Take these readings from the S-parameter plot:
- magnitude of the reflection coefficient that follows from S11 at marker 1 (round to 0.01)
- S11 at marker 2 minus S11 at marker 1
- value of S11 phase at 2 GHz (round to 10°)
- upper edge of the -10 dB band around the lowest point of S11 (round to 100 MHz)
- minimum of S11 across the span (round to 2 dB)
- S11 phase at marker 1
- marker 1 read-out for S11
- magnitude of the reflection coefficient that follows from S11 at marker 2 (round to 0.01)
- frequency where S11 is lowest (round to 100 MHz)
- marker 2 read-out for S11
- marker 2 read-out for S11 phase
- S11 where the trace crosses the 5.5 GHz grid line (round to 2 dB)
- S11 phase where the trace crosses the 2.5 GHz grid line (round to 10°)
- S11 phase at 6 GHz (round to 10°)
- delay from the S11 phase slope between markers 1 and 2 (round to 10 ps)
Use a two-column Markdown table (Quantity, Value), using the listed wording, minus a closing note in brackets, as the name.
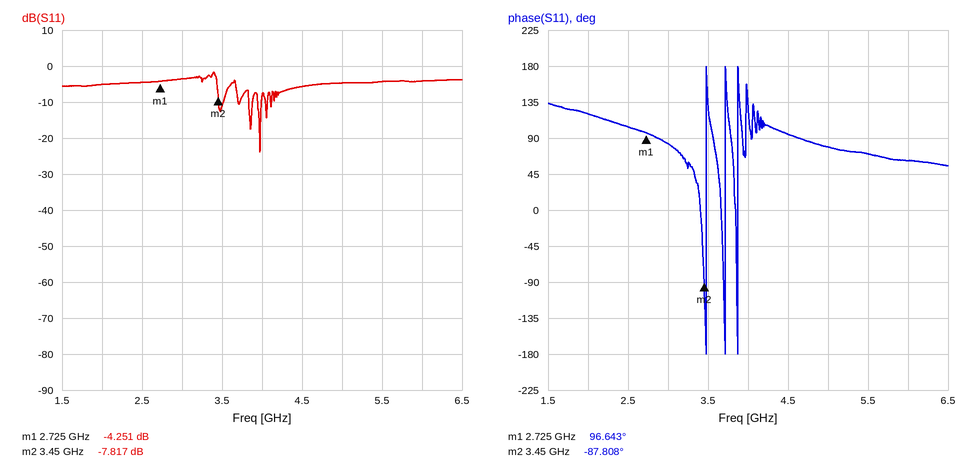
| Quantity | Value |
|---|---|
| magnitude of the reflection coefficient that follows from S11 at marker 1 | 0.61 |
| S11 at marker 2 minus S11 at marker 1 | -3.566 dB |
| value of S11 phase at 2 GHz | 120° |
| upper edge of the -10 dB band around the lowest point of S11 | 4.0 GHz |
| minimum of S11 across the span | -24 dB |
| S11 phase at marker 1 | 96.643° |
| marker 1 read-out for S11 | -4.251 dB |
| magnitude of the reflection coefficient that follows from S11 at marker 2 | 0.41 |
| frequency where S11 is lowest | 4.0 GHz |
| marker 2 read-out for S11 | -7.817 dB |
| marker 2 read-out for S11 phase | -87.808° |
| S11 where the trace crosses the 5.5 GHz grid line | -4 dB |
| S11 phase where the trace crosses the 2.5 GHz grid line | 100° |
| S11 phase at 6 GHz | 60° |
| delay from the S11 phase slope between markers 1 and 2 | 710 ps |
